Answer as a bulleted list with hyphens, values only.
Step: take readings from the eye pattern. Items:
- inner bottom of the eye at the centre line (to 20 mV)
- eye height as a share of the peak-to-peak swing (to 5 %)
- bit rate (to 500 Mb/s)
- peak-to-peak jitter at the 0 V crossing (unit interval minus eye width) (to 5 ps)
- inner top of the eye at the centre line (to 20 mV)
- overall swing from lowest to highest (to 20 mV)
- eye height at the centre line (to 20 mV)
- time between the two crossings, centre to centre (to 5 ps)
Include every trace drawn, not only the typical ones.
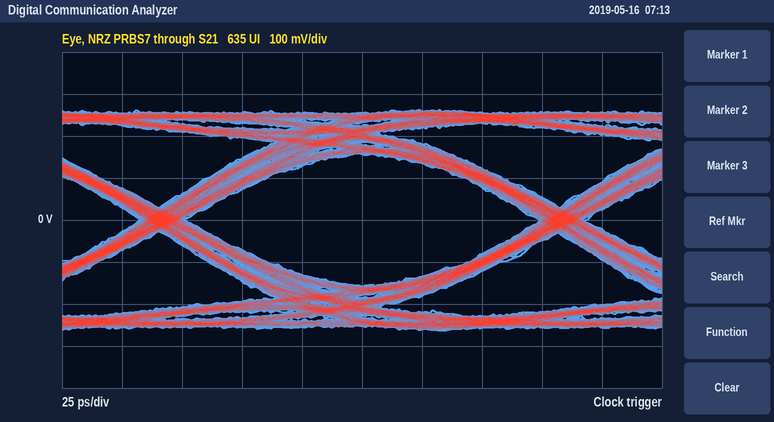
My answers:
- -160 mV
- 60 %
- 6.0 Gb/s
- 20 ps
- 160 mV
- 520 mV
- 320 mV
- 165 ps
